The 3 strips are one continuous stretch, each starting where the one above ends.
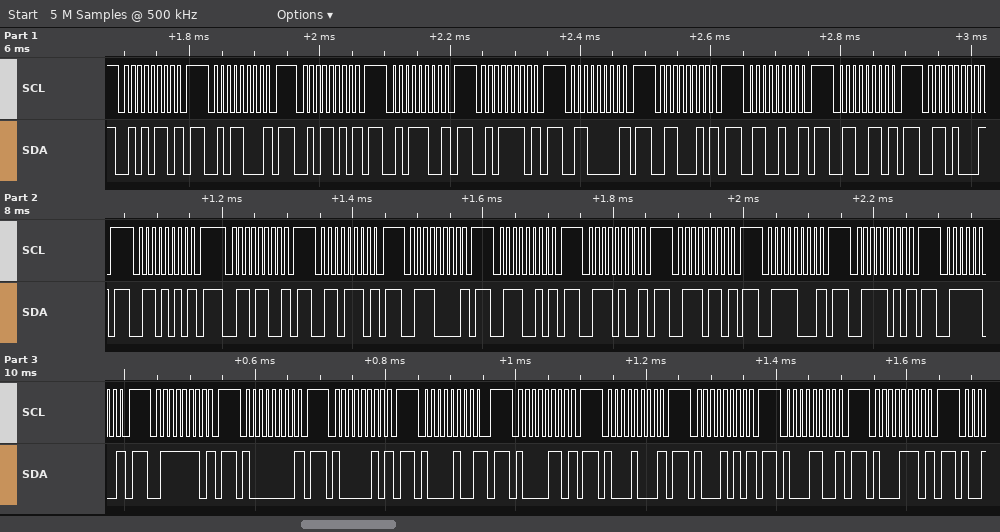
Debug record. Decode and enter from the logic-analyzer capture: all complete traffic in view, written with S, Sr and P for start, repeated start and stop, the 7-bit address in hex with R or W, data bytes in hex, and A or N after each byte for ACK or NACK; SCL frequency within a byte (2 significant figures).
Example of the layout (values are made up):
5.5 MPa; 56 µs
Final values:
S 2BW N P S 2CW N P S 2DW N P S 2EW N P S 2FW N P S 30W N P S 31W N P S 32W N P S 33W N P S 34W N P S 35W N P S 36W N P S 37W N P S 38W N P S 39W N P S 3AW N P S 3BW N P S 3CW N P S 3DW N P S 3EW N P S 3FW N P S 40W N P S 41W N P S 42W N P S 43W N P S 44W N P S 45W N P S 46W N P S 47W N P; 100 kHz
